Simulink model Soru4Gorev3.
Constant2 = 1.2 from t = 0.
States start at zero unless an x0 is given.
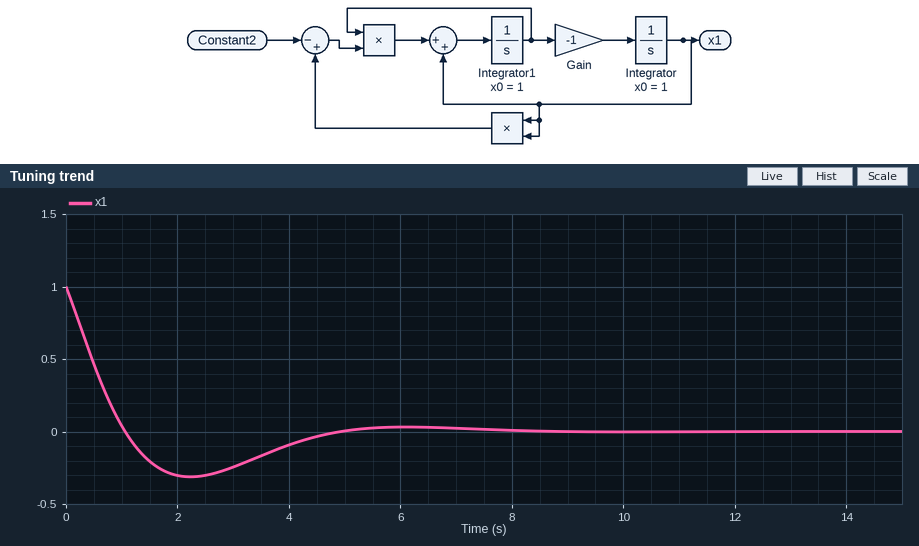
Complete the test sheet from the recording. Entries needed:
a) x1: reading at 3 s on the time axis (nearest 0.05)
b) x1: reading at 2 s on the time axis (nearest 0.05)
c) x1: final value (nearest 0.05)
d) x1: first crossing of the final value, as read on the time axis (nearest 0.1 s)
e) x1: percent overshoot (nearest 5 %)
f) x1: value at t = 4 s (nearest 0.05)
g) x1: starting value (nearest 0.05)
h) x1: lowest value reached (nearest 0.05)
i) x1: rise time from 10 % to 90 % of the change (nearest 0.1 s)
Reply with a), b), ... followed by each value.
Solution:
a) -0.25
b) -0.30
c) 0.00
d) 1.1 s
e) 30 %
f) -0.10
g) 1.00
h) -0.30
i) 0.8 s
